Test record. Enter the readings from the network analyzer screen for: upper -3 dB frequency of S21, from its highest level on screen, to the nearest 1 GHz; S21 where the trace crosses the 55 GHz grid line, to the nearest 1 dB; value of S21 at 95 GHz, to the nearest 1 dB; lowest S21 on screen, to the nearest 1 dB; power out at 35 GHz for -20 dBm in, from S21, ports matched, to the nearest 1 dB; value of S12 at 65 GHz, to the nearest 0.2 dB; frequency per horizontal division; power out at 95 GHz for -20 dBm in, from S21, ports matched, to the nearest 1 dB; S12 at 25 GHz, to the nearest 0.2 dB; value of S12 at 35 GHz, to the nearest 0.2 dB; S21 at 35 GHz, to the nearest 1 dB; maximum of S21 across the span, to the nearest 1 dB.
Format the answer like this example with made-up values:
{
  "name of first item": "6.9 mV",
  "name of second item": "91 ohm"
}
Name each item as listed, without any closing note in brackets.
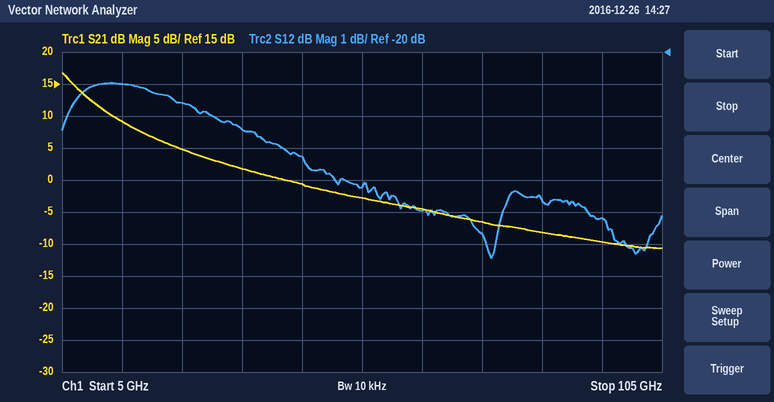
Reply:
{
  "upper -3 dB frequency of S21, from its highest level on screen, to the nearest 1 GHz": "8 GHz",
  "S21 where the trace crosses the 55 GHz grid line, to the nearest 1 dB": "-3 dB",
  "value of S21 at 95 GHz, to the nearest 1 dB": "-10 dB",
  "lowest S21 on screen, to the nearest 1 dB": "-11 dB",
  "power out at 35 GHz for -20 dBm in, from S21, ports matched, to the nearest 1 dB": "-18 dBm",
  "value of S12 at 65 GHz, to the nearest 0.2 dB": "-25.0 dB",
  "frequency per horizontal division": "10 GHz",
  "power out at 95 GHz for -20 dBm in, from S21, ports matched, to the nearest 1 dB": "-30 dBm",
  "S12 at 25 GHz, to the nearest 0.2 dB": "-21.6 dB",
  "value of S12 at 35 GHz, to the nearest 0.2 dB": "-22.4 dB",
  "S21 at 35 GHz, to the nearest 1 dB": "2 dB",
  "maximum of S21 across the span, to the nearest 1 dB": "17 dB"
}
